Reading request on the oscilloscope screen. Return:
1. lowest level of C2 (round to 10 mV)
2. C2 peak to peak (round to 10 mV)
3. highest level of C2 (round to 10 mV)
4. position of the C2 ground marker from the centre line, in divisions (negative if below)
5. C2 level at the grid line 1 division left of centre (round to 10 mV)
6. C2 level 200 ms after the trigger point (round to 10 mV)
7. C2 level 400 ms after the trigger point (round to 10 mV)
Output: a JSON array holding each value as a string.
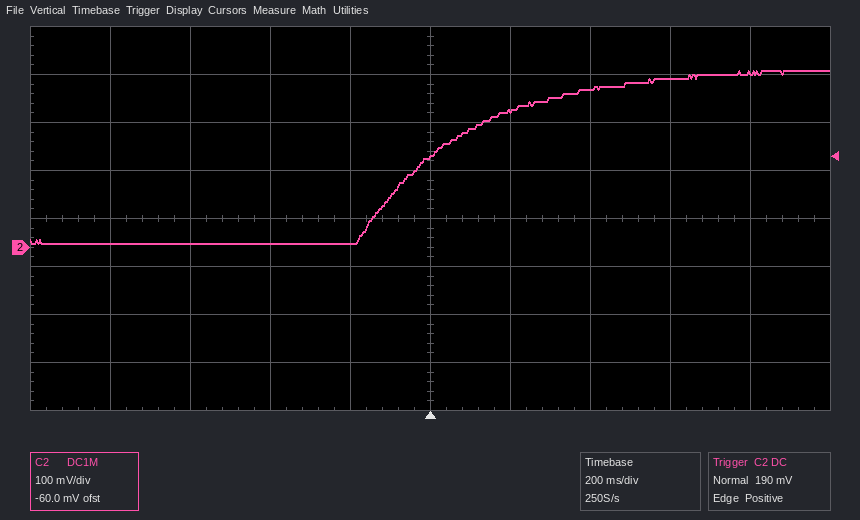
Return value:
["10 mV", "360 mV", "370 mV", "-0.6 div", "10 mV", "280 mV", "330 mV"]
